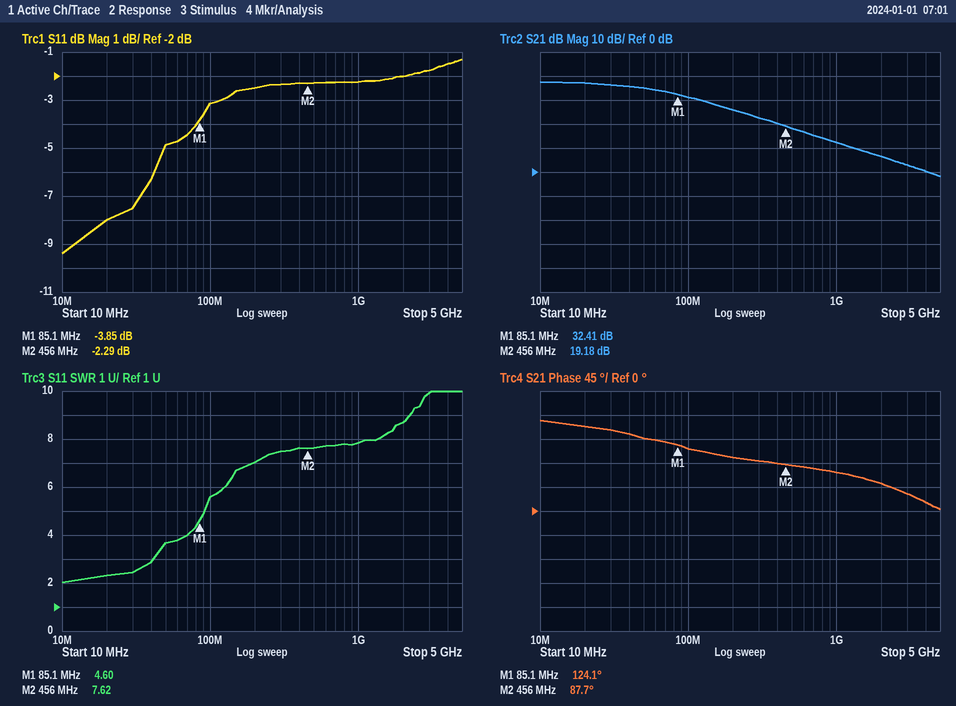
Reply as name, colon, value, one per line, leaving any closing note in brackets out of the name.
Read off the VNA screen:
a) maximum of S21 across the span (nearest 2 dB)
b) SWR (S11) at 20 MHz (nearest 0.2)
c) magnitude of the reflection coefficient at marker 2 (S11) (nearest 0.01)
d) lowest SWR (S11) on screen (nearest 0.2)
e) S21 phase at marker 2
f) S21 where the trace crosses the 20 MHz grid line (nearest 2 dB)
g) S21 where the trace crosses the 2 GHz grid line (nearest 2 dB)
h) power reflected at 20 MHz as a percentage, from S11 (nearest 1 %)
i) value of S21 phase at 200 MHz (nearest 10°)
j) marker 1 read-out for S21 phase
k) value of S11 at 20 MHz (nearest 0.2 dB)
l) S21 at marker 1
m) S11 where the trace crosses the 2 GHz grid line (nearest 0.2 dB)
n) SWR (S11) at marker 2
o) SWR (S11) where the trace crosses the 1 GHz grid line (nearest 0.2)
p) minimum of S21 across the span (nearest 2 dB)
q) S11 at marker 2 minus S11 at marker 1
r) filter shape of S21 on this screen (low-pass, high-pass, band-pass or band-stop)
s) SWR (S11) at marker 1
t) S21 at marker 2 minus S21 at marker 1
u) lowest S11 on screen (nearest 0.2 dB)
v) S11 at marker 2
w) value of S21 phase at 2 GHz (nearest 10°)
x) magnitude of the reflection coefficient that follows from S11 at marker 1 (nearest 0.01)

maximum of S21 across the span: 38 dB
SWR (S11) at 20 MHz: 2.4
magnitude of the reflection coefficient at marker 2 (S11): 0.77
lowest SWR (S11) on screen: 2.0
S21 phase at marker 2: 87.7°
S21 where the trace crosses the 20 MHz grid line: 38 dB
S21 where the trace crosses the 2 GHz grid line: 6 dB
power reflected at 20 MHz as a percentage, from S11: 16 %
value of S21 phase at 200 MHz: 100°
marker 1 read-out for S21 phase: 124.1°
value of S11 at 20 MHz: -8.0 dB
S21 at marker 1: 32.41 dB
S11 where the trace crosses the 2 GHz grid line: -2.0 dB
SWR (S11) at marker 2: 7.62
SWR (S11) where the trace crosses the 1 GHz grid line: 7.8
minimum of S21 across the span: -2 dB
S11 at marker 2 minus S11 at marker 1: 1.56 dB
filter shape of S21 on this screen: low-pass
SWR (S11) at marker 1: 4.60
S21 at marker 2 minus S21 at marker 1: -13.23 dB
lowest S11 on screen: -9.4 dB
S11 at marker 2: -2.29 dB
value of S21 phase at 2 GHz: 50°
magnitude of the reflection coefficient that follows from S11 at marker 1: 0.64
